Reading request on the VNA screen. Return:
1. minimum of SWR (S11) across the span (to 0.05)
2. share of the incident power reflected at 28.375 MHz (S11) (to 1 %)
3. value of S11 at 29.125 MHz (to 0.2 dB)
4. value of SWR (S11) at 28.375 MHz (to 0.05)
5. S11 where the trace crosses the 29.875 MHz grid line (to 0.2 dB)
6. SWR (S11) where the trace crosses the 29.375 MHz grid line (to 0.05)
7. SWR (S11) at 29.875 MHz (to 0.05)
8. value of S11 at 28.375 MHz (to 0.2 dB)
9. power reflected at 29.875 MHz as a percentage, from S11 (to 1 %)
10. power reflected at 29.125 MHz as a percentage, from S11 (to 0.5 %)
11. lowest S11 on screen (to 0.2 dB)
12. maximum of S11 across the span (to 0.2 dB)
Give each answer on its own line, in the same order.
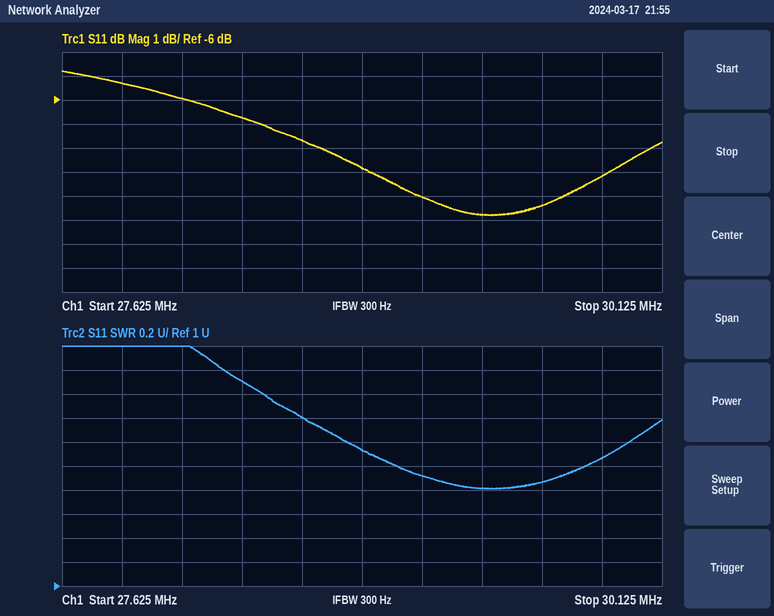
1.80
21 %
-10.0 dB
2.70
-9.2 dB
1.80
2.05
-6.8 dB
12 %
10.0 %
-10.8 dB
-4.8 dB
